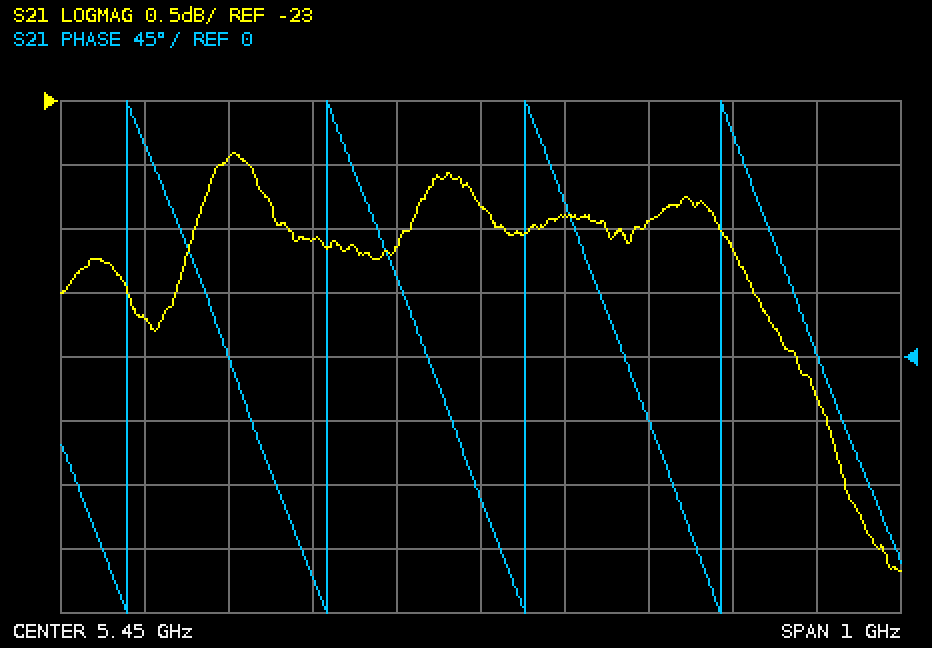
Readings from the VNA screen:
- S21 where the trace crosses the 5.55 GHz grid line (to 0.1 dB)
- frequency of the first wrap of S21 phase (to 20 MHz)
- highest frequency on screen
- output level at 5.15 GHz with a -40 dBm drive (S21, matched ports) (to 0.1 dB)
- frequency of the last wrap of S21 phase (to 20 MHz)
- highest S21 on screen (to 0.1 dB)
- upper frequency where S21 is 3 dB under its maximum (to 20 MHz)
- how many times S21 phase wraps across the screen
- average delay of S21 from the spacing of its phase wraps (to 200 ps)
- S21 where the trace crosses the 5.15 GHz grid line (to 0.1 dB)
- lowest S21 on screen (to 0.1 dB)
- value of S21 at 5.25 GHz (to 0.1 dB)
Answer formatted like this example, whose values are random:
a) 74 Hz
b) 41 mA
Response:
a) -23.9 dB
b) 5.02 GHz
c) 5.95 GHz
d) -63.4 dBm
e) 5.74 GHz
f) -23.4 dB
g) 5.92 GHz
h) 4
i) 4.2 ns
j) -23.4 dB
k) -26.7 dB
l) -24.1 dB
